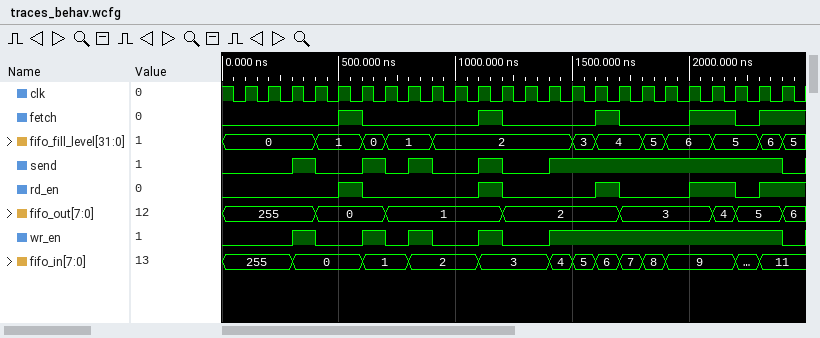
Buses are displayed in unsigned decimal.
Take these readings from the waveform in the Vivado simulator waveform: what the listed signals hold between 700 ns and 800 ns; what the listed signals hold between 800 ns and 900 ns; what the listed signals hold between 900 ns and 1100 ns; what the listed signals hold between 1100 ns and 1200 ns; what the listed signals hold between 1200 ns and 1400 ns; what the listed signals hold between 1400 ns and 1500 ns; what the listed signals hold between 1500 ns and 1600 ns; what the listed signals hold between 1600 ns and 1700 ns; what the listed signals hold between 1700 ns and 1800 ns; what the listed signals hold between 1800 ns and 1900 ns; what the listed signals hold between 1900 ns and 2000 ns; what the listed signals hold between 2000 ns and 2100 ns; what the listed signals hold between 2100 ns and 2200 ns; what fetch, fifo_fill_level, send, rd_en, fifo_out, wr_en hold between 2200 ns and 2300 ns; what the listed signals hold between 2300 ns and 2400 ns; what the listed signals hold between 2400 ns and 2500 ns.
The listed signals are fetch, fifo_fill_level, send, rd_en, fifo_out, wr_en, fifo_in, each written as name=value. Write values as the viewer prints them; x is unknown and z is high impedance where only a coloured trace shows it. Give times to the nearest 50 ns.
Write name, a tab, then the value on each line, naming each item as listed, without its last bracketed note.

what the listed signals hold between 700 ns and 800 ns	fetch=0, fifo_fill_level=1, send=0, rd_en=0, fifo_out=1, wr_en=0, fifo_in=1
what the listed signals hold between 800 ns and 900 ns	fetch=0, fifo_fill_level=1, send=1, rd_en=0, fifo_out=1, wr_en=1, fifo_in=2
what the listed signals hold between 900 ns and 1100 ns	fetch=0, fifo_fill_level=2, send=0, rd_en=0, fifo_out=1, wr_en=0, fifo_in=2
what the listed signals hold between 1100 ns and 1200 ns	fetch=1, fifo_fill_level=2, send=1, rd_en=1, fifo_out=1, wr_en=1, fifo_in=3
what the listed signals hold between 1200 ns and 1400 ns	fetch=0, fifo_fill_level=2, send=0, rd_en=0, fifo_out=2, wr_en=0, fifo_in=3
what the listed signals hold between 1400 ns and 1500 ns	fetch=0, fifo_fill_level=2, send=1, rd_en=0, fifo_out=2, wr_en=1, fifo_in=4
what the listed signals hold between 1500 ns and 1600 ns	fetch=0, fifo_fill_level=3, send=1, rd_en=0, fifo_out=2, wr_en=1, fifo_in=5
what the listed signals hold between 1600 ns and 1700 ns	fetch=1, fifo_fill_level=4, send=1, rd_en=1, fifo_out=2, wr_en=1, fifo_in=6
what the listed signals hold between 1700 ns and 1800 ns	fetch=0, fifo_fill_level=4, send=1, rd_en=0, fifo_out=3, wr_en=1, fifo_in=7
what the listed signals hold between 1800 ns and 1900 ns	fetch=0, fifo_fill_level=5, send=1, rd_en=0, fifo_out=3, wr_en=1, fifo_in=8
what the listed signals hold between 1900 ns and 2000 ns	fetch=0, fifo_fill_level=6, send=1, rd_en=0, fifo_out=3, wr_en=1, fifo_in=9
what the listed signals hold between 2000 ns and 2100 ns	fetch=1, fifo_fill_level=6, send=1, rd_en=1, fifo_out=3, wr_en=1, fifo_in=9
what the listed signals hold between 2100 ns and 2200 ns	fetch=1, fifo_fill_level=5, send=1, rd_en=1, fifo_out=4, wr_en=1, fifo_in=9
what fetch, fifo_fill_level, send, rd_en, fifo_out, wr_en hold between 2200 ns and 2300 ns	fetch=0, fifo_fill_level=5, send=1, rd_en=0, fifo_out=5, wr_en=1
what the listed signals hold between 2300 ns and 2400 ns	fetch=1, fifo_fill_level=6, send=1, rd_en=1, fifo_out=5, wr_en=1, fifo_in=11
what the listed signals hold between 2400 ns and 2500 ns	fetch=1, fifo_fill_level=5, send=0, rd_en=1, fifo_out=6, wr_en=0, fifo_in=11
